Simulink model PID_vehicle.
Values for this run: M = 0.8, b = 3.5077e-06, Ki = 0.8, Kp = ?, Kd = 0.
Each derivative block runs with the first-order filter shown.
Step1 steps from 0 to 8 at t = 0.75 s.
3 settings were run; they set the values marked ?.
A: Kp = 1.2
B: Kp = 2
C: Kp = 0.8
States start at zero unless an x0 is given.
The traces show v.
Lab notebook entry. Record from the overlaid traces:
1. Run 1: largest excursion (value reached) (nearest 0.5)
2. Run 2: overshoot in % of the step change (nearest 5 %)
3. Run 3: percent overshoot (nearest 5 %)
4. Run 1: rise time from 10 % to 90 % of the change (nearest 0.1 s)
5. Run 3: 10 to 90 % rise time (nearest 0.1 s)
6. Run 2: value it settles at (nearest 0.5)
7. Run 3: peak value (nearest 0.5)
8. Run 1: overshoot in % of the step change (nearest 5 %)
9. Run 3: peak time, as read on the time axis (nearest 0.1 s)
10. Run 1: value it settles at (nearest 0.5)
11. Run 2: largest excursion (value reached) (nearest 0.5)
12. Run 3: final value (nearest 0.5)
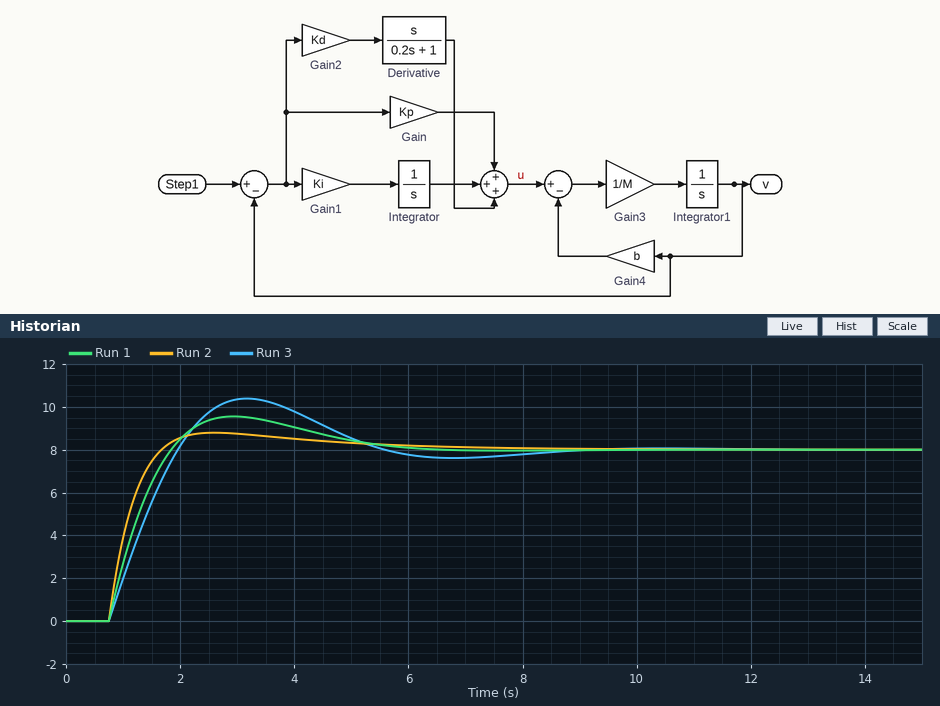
9.5
10 %
30 %
0.8 s
0.9 s
8.0
10.5
20 %
3.2 s
8.0
9.0
8.0
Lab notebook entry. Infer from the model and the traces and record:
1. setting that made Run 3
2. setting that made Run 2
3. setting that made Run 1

C
B
A
